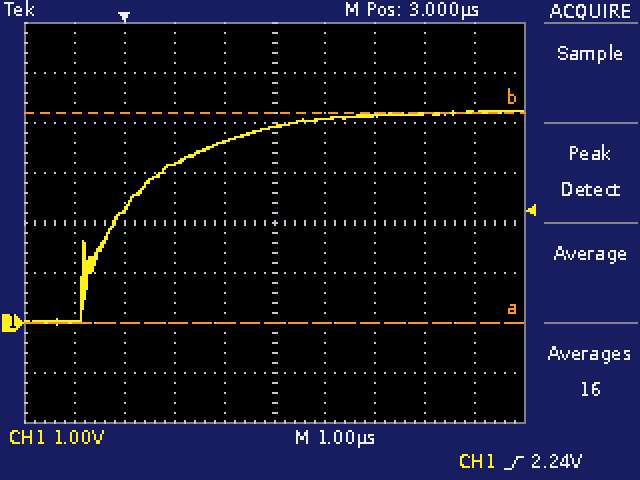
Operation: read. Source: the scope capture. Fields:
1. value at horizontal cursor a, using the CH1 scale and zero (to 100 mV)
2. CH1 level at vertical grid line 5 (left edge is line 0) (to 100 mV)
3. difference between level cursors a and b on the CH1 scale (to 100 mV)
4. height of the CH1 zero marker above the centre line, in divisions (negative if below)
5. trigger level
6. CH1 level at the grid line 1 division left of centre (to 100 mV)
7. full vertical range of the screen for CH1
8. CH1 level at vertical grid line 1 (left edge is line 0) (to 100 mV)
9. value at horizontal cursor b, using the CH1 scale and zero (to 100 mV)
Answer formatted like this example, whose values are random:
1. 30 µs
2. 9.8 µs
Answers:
1. 0.0 V
2. 3.9 V
3. 4.2 V
4. -2.0 div
5. 2.24 V
6. 3.6 V
7. 8 V
8. 0.0 V
9. 4.2 V
